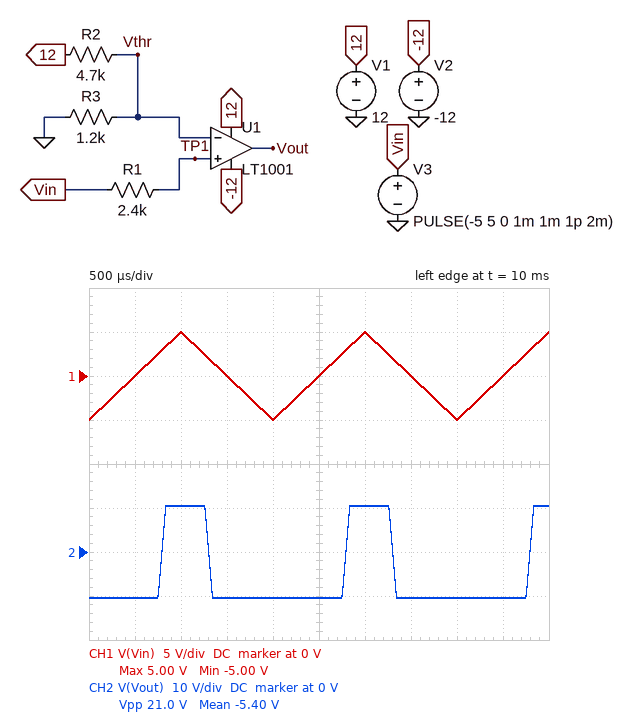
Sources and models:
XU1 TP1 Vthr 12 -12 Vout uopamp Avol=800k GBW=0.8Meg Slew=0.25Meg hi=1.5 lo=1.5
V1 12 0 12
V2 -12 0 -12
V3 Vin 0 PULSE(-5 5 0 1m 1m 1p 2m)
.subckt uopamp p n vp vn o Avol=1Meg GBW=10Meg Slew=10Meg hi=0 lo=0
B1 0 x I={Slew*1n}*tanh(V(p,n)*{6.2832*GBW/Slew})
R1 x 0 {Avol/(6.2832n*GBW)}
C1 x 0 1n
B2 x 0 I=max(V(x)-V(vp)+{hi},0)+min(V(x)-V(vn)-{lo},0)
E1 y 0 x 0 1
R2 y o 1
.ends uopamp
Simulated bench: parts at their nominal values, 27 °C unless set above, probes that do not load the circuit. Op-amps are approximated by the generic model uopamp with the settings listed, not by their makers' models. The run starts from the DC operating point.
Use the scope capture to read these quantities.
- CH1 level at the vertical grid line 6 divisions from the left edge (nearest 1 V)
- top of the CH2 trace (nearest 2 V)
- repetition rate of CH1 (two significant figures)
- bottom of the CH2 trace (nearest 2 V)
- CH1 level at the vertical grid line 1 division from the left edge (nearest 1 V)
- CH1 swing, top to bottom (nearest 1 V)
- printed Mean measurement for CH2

5 V
10 V
500 Hz
-10 V
0 V
10 V
-5.40 V
